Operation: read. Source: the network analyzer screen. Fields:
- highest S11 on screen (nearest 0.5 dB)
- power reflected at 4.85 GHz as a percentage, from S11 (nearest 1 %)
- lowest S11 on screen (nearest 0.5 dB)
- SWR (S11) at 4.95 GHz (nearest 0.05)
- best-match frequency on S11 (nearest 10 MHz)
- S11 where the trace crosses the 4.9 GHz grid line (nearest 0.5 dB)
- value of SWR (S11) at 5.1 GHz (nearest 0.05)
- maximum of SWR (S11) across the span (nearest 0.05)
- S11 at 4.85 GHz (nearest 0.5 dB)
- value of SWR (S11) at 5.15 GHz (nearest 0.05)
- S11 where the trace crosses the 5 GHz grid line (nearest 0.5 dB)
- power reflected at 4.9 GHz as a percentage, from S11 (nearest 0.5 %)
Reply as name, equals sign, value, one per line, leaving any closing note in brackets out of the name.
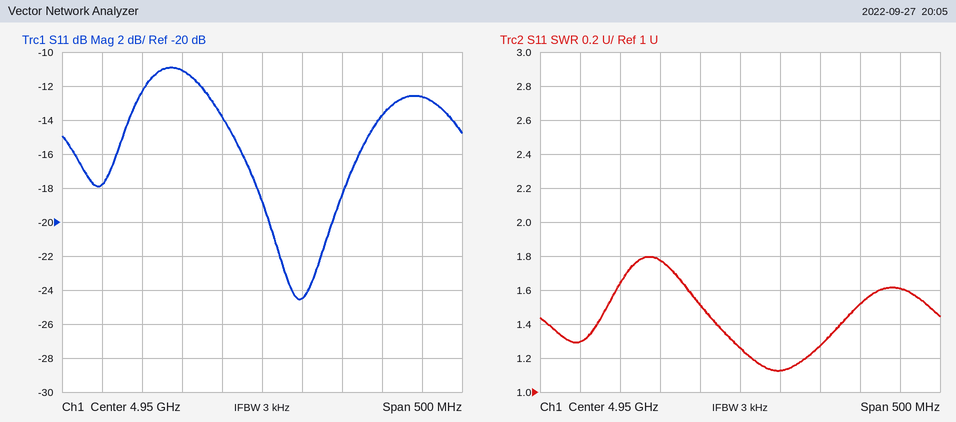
highest S11 on screen = -11.0 dB
power reflected at 4.85 GHz as a percentage, from S11 = 8 %
lowest S11 on screen = -24.5 dB
SWR (S11) at 4.95 GHz = 1.25
best-match frequency on S11 = 5.00 GHz
S11 where the trace crosses the 4.9 GHz grid line = -14.0 dB
value of SWR (S11) at 5.1 GHz = 1.50
maximum of SWR (S11) across the span = 1.80
S11 at 4.85 GHz = -11.0 dB
value of SWR (S11) at 5.15 GHz = 1.60
S11 where the trace crosses the 5 GHz grid line = -24.5 dB
power reflected at 4.9 GHz as a percentage, from S11 = 4.0 %
